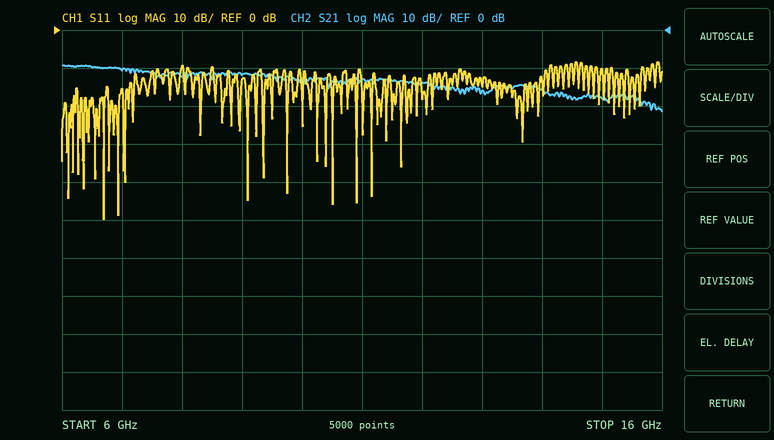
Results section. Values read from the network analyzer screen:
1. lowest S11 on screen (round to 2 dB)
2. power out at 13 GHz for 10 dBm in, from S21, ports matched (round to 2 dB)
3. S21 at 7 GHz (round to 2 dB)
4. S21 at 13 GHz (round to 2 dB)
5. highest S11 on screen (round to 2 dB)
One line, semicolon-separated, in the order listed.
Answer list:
-50 dB; -6 dBm; -10 dB; -16 dB; -8 dB
